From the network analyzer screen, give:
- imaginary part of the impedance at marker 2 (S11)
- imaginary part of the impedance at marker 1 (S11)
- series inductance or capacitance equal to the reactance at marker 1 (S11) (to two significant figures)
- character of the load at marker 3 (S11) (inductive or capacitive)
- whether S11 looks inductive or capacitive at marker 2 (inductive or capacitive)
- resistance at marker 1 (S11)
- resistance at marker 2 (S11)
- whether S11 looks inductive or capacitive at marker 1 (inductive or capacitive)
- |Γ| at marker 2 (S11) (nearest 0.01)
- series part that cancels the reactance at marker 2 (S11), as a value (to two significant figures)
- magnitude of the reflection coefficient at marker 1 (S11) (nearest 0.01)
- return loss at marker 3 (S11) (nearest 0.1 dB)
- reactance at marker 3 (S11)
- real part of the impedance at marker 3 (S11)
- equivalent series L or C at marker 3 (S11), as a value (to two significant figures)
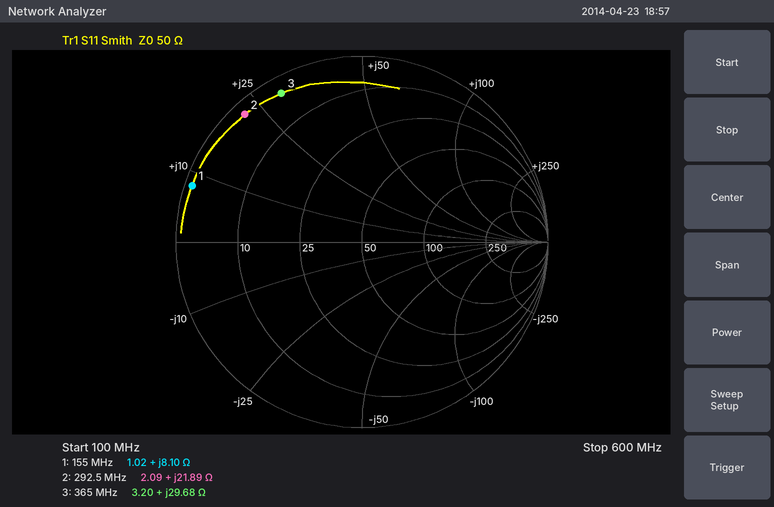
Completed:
+21.89 Ω
+8.10 Ω
8.3 nH
inductive
inductive
1.02 Ω
2.09 Ω
inductive
0.93
25 pF
0.96
0.8 dB
+29.68 Ω
3.20 Ω
13 nH
